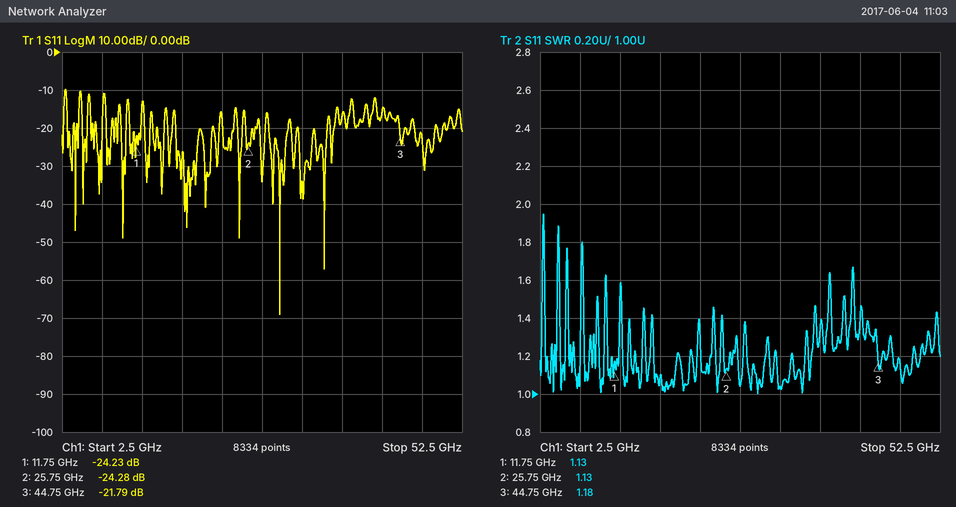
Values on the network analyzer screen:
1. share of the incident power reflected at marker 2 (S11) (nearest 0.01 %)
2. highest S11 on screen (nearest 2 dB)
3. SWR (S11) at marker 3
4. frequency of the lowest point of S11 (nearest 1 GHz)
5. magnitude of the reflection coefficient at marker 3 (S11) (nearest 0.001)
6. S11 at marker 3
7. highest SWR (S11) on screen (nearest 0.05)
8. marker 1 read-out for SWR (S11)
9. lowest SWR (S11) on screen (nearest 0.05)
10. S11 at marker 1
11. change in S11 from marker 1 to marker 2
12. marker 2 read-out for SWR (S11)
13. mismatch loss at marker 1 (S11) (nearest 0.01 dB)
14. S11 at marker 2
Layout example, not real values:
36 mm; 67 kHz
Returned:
0.37 %; -10 dB; 1.18; 30 GHz; 0.081; -21.79 dB; 1.95; 1.13; 1.00; -24.23 dB; -0.05 dB; 1.13; 0.02 dB; -24.28 dB
